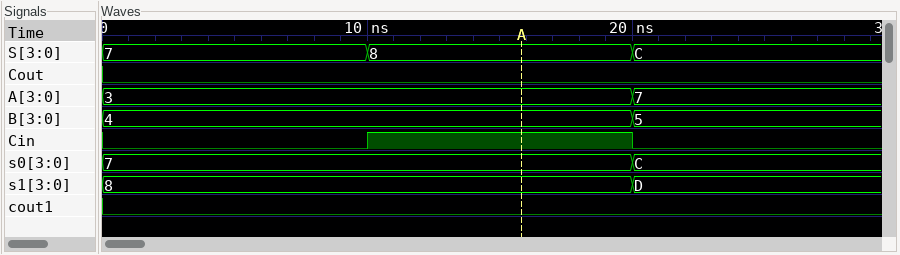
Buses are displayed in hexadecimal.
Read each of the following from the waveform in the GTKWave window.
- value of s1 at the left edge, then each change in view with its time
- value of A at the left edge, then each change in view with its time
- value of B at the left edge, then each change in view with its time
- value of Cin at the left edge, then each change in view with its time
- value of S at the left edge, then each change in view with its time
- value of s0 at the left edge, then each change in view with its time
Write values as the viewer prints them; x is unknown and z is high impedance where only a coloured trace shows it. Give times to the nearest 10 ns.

8, D at 20 ns
3, 7 at 20 ns
4, 5 at 20 ns
0, 1 at 10 ns, 0 at 20 ns
7, 8 at 10 ns, C at 20 ns
7, C at 20 ns
